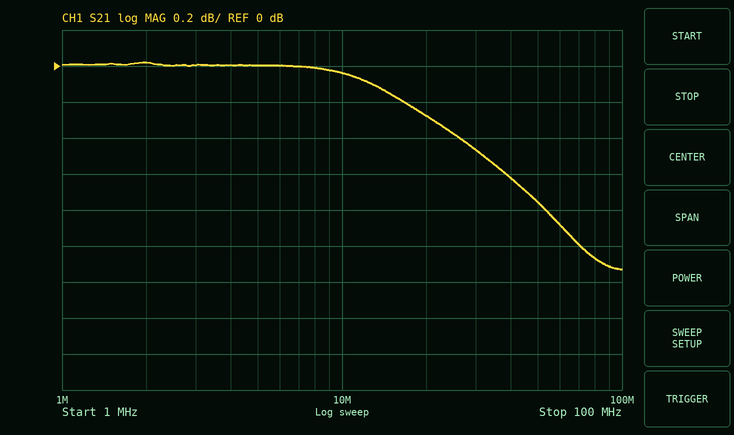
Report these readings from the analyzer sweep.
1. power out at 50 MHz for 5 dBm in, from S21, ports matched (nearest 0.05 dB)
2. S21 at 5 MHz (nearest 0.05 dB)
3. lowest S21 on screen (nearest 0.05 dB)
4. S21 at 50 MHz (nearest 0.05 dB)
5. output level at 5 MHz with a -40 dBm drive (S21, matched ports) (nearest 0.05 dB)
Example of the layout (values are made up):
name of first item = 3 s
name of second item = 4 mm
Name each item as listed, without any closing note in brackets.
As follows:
power out at 50 MHz for 5 dBm in, from S21, ports matched = 4.25 dBm
S21 at 5 MHz = 0.00 dB
lowest S21 on screen = -1.15 dB
S21 at 50 MHz = -0.75 dB
output level at 5 MHz with a -40 dBm drive (S21, matched ports) = -40.00 dBm
